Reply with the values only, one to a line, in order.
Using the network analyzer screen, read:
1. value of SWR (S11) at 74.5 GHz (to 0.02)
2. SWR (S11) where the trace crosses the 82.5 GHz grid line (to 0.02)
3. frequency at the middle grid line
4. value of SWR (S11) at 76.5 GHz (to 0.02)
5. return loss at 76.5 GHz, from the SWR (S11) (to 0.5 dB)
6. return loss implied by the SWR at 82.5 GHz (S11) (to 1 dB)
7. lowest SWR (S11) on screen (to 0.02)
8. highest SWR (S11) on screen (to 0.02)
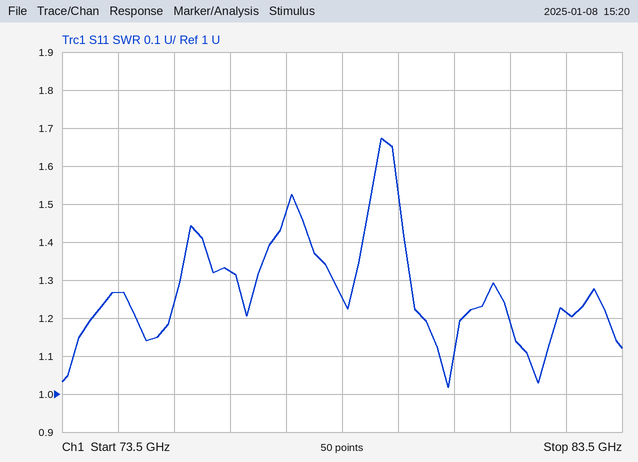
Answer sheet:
1.26
1.22
78.5 GHz
1.32
17.0 dB
20 dB
1.02
1.68
